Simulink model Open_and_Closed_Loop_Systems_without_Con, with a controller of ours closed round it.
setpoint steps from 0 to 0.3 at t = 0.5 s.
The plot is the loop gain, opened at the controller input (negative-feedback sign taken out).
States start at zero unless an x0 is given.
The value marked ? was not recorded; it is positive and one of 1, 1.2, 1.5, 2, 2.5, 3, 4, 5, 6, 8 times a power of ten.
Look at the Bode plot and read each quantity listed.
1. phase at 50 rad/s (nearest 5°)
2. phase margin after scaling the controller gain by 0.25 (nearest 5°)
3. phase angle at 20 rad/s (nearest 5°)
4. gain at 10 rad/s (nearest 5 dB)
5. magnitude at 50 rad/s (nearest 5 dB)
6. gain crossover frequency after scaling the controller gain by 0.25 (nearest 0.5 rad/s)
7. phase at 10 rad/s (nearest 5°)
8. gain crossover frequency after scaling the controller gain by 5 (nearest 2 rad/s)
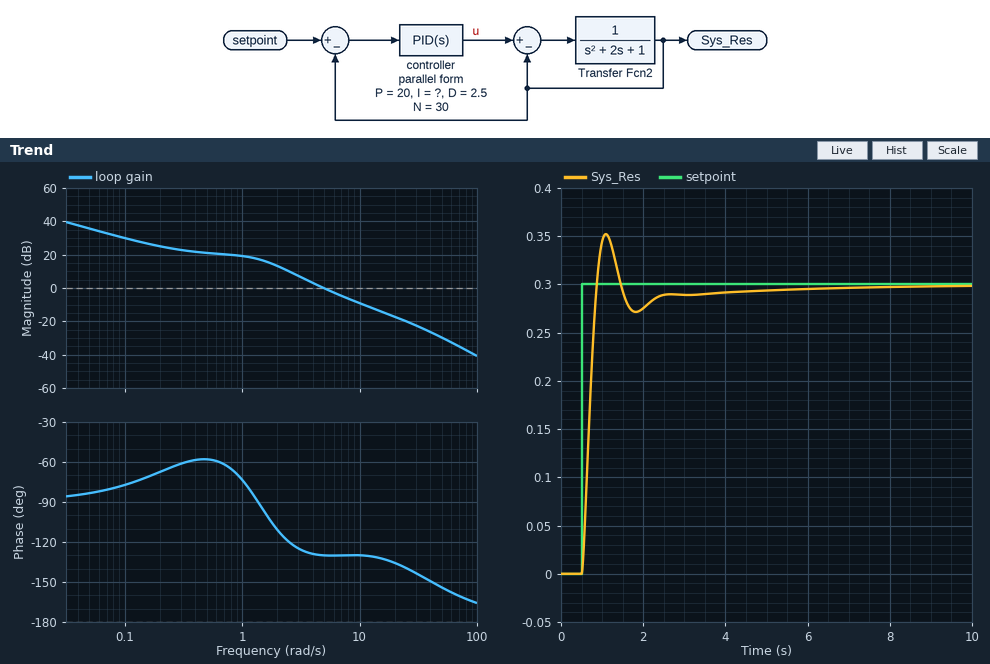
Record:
-155°
65°
-135°
-10 dB
-30 dB
2.0 rad/s
-130°
16 rad/s
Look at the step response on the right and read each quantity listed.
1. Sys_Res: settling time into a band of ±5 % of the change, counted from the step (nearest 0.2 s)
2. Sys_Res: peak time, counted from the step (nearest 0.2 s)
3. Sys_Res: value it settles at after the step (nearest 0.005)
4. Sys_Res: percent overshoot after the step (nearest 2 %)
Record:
1.8 s
0.6 s
0.300
18 %
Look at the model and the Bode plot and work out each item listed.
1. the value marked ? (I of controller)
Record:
6
